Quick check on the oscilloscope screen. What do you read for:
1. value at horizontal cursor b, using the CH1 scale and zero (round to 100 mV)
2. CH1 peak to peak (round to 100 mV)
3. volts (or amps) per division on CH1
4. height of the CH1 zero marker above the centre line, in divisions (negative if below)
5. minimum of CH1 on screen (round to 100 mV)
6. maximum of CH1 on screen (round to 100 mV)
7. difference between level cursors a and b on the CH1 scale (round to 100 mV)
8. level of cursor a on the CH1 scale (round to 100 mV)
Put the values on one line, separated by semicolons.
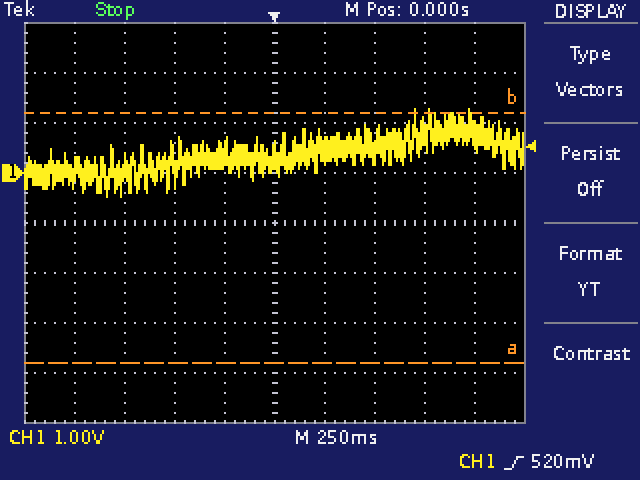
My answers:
1.2 V; 1.8 V; 1 V; +1.0 div; -500 mV; 1.3 V; 5.0 V; -3.8 V
